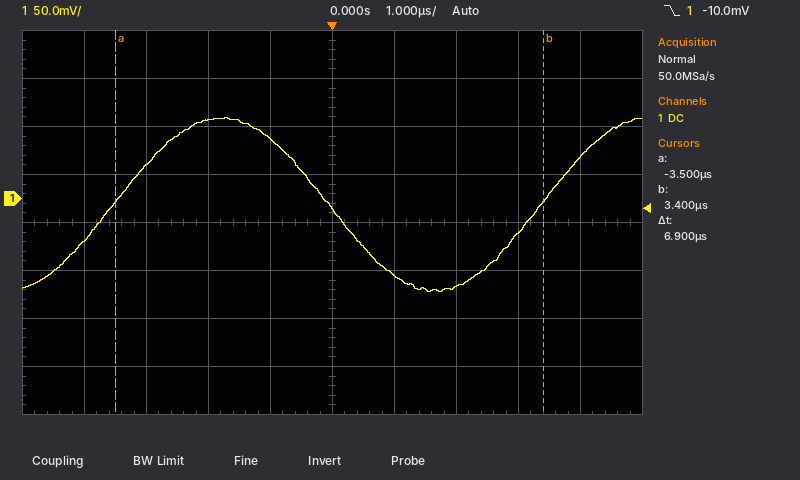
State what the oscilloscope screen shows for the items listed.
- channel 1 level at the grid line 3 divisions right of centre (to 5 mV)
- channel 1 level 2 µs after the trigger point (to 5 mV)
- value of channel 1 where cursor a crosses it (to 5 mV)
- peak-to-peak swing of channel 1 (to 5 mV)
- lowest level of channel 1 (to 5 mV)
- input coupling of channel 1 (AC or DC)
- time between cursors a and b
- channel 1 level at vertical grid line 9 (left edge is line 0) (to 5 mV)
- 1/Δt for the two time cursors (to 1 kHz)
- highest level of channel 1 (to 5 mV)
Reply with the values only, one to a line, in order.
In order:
-35 mV
-90 mV
-5 mV
180 mV
-95 mV
DC
6.9 µs
45 mV
145 kHz
85 mV
